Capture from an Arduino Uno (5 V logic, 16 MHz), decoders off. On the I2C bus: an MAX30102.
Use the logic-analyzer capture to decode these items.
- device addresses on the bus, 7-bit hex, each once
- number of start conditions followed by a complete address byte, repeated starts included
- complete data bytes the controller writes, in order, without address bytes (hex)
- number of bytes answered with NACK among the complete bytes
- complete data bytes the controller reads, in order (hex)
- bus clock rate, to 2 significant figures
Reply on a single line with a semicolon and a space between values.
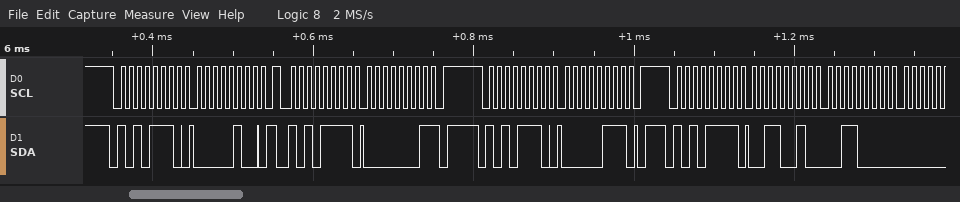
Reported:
0x57; 4; 04 07; 1; 01 32 30; 100 kHz
